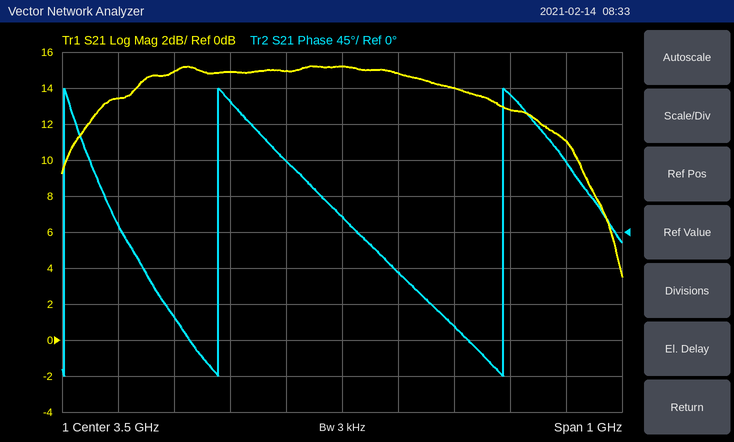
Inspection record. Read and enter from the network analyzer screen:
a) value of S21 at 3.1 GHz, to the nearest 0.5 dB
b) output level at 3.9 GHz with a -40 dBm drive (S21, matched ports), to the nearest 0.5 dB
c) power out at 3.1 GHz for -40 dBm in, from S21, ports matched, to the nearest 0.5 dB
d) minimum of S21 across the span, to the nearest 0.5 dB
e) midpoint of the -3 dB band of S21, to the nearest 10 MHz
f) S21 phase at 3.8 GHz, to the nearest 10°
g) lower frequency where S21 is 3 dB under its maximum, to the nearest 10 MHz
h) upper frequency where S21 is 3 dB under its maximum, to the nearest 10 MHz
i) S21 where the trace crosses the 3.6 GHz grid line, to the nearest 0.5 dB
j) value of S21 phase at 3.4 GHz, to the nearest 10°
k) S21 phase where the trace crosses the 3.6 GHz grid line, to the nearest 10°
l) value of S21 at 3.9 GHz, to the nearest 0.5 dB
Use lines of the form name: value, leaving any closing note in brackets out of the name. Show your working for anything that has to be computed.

value of S21 at 3.1 GHz, to the nearest 0.5 dB: 13.5 dB
output level at 3.9 GHz with a -40 dBm drive (S21, matched ports), to the nearest 0.5 dB: -40 dBm + (11.0 dB) = -29.0 dBm
power out at 3.1 GHz for -40 dBm in, from S21, ports matched, to the nearest 0.5 dB: -40 dBm + (13.5 dB) = -26.5 dBm
minimum of S21 across the span, to the nearest 0.5 dB: 3.5 dB
midpoint of the -3 dB band of S21, to the nearest 10 MHz: 3.45 GHz
S21 phase at 3.8 GHz, to the nearest 10°: 170°
lower frequency where S21 is 3 dB under its maximum, to the nearest 10 MHz: 3.05 GHz
upper frequency where S21 is 3 dB under its maximum, to the nearest 10 MHz: 3.85 GHz
S21 where the trace crosses the 3.6 GHz grid line, to the nearest 0.5 dB: 15.0 dB
value of S21 phase at 3.4 GHz, to the nearest 10°: 90°
S21 phase where the trace crosses the 3.6 GHz grid line, to the nearest 10°: -50°
value of S21 at 3.9 GHz, to the nearest 0.5 dB: 11.0 dB
